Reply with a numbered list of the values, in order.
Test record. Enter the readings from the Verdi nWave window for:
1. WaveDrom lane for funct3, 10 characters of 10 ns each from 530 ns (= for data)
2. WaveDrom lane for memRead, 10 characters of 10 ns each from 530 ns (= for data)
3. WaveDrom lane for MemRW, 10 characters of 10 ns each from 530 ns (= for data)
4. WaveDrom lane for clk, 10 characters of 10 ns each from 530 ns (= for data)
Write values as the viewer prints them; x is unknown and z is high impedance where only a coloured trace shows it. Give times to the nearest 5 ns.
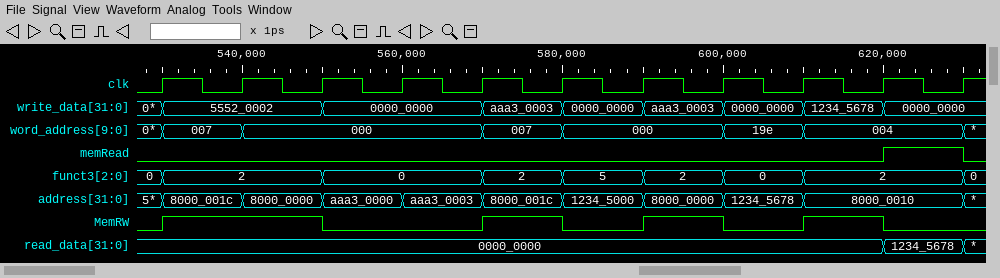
1. {name: 'funct3', wave: '=.=.=====.', data: '2 0 2 5 2 0 2'}
2. {name: 'memRead', wave: '0........1'}
3. {name: 'MemRW', wave: '1.0.101010'}
4. {name: 'clk', wave: 'p.........'}
